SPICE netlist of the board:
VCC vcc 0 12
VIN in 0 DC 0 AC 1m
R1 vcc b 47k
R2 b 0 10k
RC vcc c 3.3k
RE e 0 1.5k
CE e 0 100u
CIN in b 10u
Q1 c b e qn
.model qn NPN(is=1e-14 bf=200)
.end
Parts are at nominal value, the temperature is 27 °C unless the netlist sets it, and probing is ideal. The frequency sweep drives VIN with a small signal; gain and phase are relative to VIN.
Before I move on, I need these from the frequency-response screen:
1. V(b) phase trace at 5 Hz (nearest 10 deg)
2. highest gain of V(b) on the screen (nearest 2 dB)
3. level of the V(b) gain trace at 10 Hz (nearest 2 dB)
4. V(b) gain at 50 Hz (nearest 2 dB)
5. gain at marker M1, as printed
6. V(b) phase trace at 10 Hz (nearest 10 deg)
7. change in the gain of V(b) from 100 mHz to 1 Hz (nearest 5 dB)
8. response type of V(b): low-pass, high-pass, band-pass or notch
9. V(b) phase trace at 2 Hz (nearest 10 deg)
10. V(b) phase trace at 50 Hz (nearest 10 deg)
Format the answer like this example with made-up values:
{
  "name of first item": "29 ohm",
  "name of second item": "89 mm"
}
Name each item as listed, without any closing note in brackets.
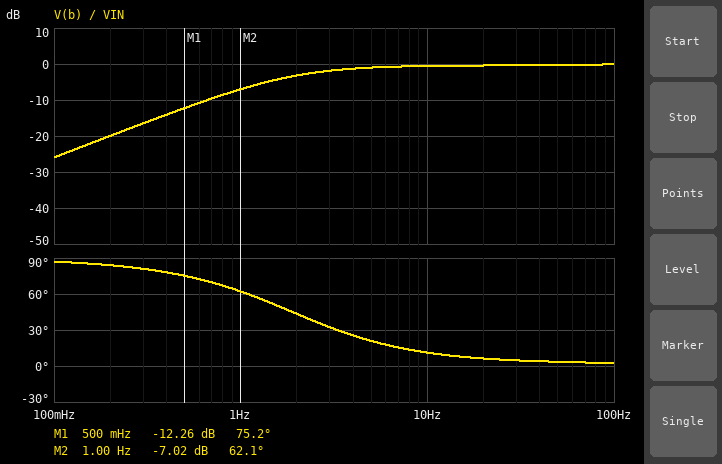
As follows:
{
  "V(b) phase trace at 5 Hz": "20 deg",
  "highest gain of V(b) on the screen": "0 dB",
  "level of the V(b) gain trace at 10 Hz": "0 dB",
  "V(b) gain at 50 Hz": "0 dB",
  "gain at marker M1, as printed": "-12.26 dB",
  "V(b) phase trace at 10 Hz": "10 deg",
  "change in the gain of V(b) from 100 mHz to 1 Hz": "20 dB",
  "response type of V(b): low-pass, high-pass, band-pass or notch": "high-pass",
  "V(b) phase trace at 2 Hz": "40 deg",
  "V(b) phase trace at 50 Hz": "0 deg"
}
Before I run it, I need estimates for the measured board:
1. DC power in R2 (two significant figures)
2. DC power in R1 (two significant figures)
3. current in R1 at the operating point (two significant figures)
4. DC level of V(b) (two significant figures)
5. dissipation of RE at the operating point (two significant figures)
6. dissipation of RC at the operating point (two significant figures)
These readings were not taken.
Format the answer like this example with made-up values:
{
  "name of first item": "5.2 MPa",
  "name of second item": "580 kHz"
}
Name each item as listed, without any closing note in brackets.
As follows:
{
  "DC power in R2": "430 µW",
  "DC power in R1": "2.1 mW",
  "current in R1 at the operating point": "210 µA",
  "DC level of V(b)": "2.1 V",
  "dissipation of RE at the operating point": "1.3 mW",
  "dissipation of RC at the operating point": "2.9 mW"
}
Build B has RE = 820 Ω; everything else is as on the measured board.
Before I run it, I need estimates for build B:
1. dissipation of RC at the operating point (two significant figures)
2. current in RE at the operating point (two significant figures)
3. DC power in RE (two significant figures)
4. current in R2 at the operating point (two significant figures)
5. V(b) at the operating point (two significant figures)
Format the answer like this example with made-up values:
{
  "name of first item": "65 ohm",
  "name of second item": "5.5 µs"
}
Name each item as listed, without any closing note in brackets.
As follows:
{
  "dissipation of RC at the operating point": "9.1 mW",
  "current in RE at the operating point": "1.7 mA",
  "DC power in RE": "2.3 mW",
  "current in R2 at the operating point": "200 µA",
  "V(b) at the operating point": "2.0 V"
}
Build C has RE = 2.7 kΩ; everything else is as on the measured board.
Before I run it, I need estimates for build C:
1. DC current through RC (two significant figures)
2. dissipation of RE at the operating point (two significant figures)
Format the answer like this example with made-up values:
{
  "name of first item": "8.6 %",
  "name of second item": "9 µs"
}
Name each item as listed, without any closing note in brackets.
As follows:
{
  "DC current through RC": "530 µA",
  "dissipation of RE at the operating point": "770 µW"
}
